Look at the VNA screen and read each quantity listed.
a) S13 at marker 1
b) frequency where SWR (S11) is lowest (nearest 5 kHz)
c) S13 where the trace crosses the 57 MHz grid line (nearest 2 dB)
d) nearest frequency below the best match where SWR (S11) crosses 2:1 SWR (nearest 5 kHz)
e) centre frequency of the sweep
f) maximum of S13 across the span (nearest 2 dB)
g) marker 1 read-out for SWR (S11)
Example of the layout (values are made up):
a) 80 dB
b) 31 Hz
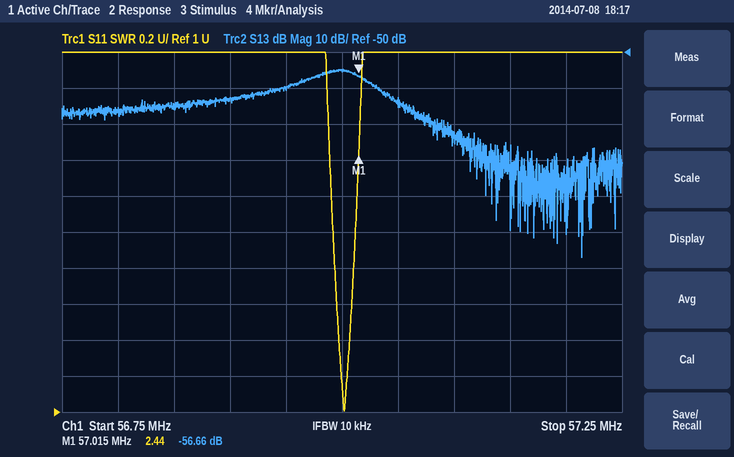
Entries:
a) -56.66 dB
b) 57.000 MHz
c) -56 dB
d) 56.990 MHz
e) 57 MHz
f) -54 dB
g) 2.44
